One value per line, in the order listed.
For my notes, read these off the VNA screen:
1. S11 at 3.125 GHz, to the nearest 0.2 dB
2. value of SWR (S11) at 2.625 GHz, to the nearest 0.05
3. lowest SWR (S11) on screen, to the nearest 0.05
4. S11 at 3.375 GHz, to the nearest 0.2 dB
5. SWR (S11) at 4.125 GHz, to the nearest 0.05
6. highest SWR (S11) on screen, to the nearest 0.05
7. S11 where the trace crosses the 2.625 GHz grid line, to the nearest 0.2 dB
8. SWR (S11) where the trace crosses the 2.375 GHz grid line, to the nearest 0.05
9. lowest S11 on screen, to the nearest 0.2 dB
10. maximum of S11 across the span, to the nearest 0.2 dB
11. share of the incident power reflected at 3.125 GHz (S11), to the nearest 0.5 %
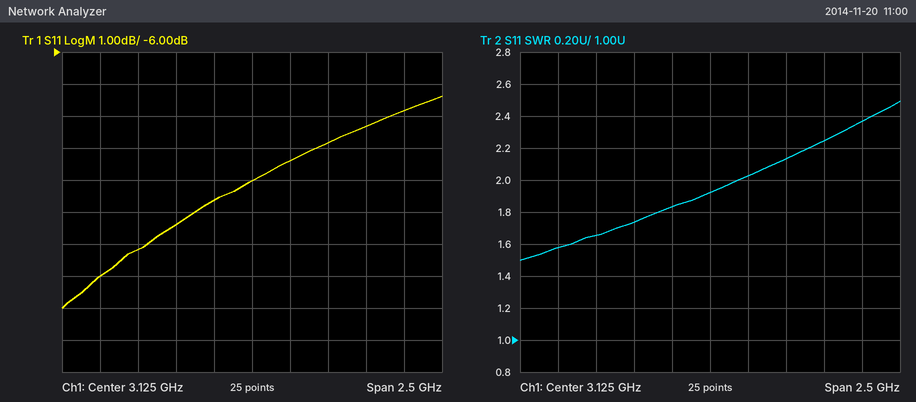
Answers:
-10.0 dB
1.75
1.50
-9.4 dB
2.35
2.50
-11.4 dB
1.65
-14.0 dB
-7.4 dB
10.0 %
